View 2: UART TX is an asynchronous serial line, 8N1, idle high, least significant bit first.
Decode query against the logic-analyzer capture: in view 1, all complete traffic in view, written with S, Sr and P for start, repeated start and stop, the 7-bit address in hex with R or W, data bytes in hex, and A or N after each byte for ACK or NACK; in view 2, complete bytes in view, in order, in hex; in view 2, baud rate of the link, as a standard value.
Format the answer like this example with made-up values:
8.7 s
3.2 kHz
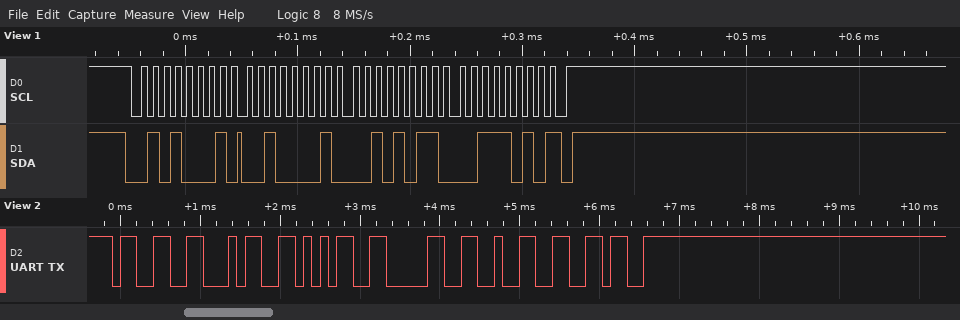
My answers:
S 28R A 21 A 2B A 3A N P
33 34 35 30 32 36
9600 baud
